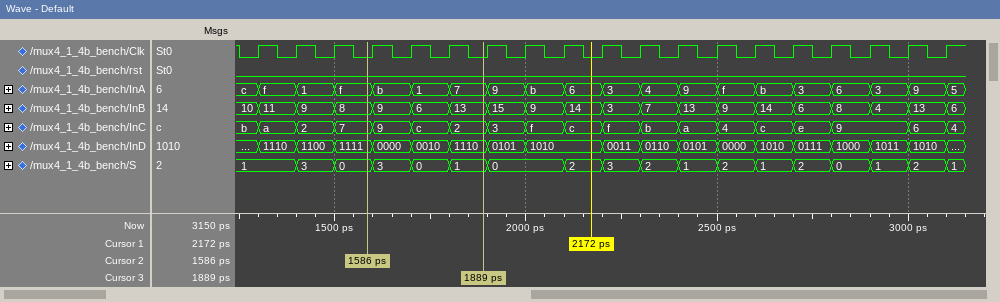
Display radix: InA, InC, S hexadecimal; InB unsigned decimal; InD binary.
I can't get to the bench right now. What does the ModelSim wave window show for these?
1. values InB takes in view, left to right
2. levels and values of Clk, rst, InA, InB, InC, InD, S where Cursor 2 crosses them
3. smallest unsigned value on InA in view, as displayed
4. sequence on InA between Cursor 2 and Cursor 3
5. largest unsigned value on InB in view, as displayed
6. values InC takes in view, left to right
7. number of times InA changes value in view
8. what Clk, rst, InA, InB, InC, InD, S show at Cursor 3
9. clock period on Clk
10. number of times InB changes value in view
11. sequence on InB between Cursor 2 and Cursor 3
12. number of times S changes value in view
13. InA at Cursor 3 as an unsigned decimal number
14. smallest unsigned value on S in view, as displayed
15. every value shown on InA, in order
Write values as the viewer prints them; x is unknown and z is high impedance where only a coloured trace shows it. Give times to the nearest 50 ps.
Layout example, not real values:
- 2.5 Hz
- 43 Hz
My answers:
- 10, 11, 9, 8, 9, 6, 13, 15, 9, 14, 3, 7, 13, 9, 14, 6, 8, 4, 13, 6
- Clk=0, rst=0, InA=f, InB=8, InC=7, InD=1111, S=0
- 1
- f, b, 1, 7
- 15
- b, a, 2, 7, 9, c, 2, 3, f, c, f, b, a, 4, c, e, 9, 6, 4
- 19
- Clk=0, rst=0, InA=7, InB=13, InC=2, InD=1110, S=1
- 100 ps
- 19
- 8, 9, 6, 13
- 17
- 7
- 0
- c, f, 1, f, b, 1, 7, 9, b, 6, 3, 4, 9, f, b, 3, 6, 3, 9, 5
